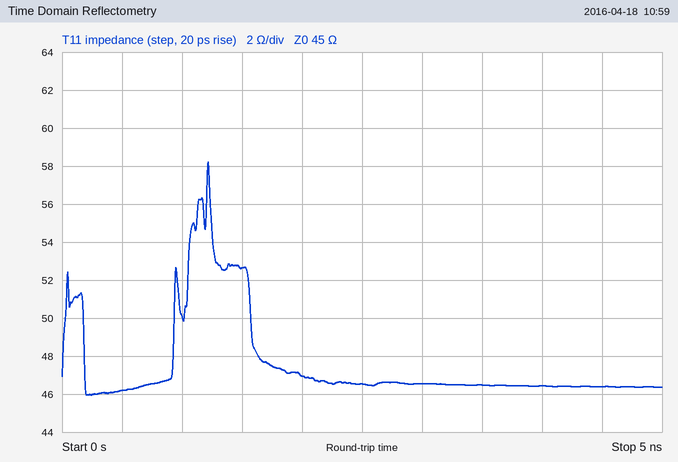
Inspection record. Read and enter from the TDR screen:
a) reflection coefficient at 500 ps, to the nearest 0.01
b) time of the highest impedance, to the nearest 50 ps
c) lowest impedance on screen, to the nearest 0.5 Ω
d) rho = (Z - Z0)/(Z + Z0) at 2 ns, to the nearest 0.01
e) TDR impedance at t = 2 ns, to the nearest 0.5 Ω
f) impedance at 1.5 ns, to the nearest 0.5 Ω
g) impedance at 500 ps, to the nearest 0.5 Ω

+0.01
1.20 ns
46.0 Ω
+0.02
47.0 Ω
52.5 Ω
46.0 Ω
